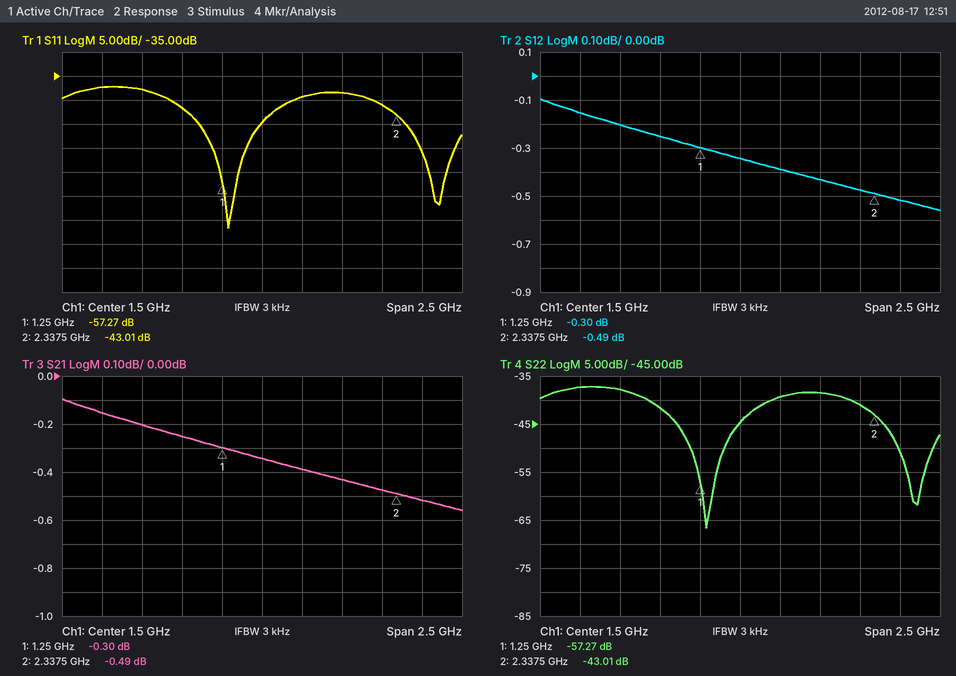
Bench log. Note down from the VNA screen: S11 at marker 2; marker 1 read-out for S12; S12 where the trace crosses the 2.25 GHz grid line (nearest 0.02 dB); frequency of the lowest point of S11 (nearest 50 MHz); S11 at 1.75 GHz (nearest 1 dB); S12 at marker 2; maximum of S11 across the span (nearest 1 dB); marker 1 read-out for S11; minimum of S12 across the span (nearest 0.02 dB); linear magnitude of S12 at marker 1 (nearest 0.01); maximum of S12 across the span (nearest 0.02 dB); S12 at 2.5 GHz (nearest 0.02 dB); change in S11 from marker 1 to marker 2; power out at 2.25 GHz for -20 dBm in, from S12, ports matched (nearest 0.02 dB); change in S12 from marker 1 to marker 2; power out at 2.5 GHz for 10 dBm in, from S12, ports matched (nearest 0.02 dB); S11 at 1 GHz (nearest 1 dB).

-43.01 dB
-0.30 dB
-0.48 dB
1.30 GHz
-39 dB
-0.49 dB
-37 dB
-57.27 dB
-0.56 dB
0.97
-0.10 dB
-0.52 dB
14.26 dB
-20.48 dBm
-0.19 dB
9.48 dBm
-42 dB
